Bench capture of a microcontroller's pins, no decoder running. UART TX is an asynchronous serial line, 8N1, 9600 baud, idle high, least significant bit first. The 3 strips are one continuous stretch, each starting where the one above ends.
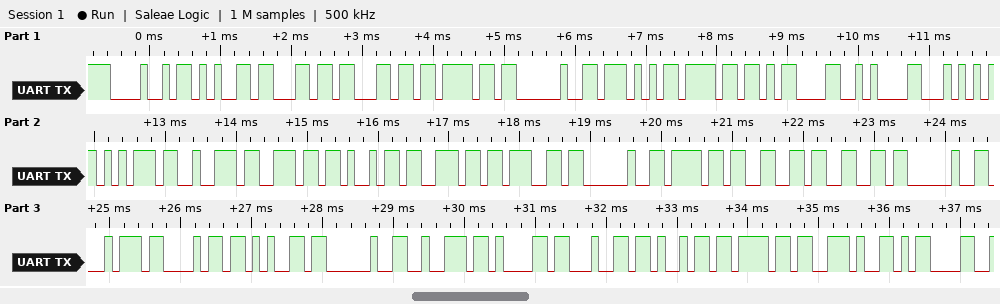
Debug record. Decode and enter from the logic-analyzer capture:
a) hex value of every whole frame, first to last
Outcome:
48 65 6C 6C 6F 20 57 6F 0D 0A 54 75 72 6E 69 6E 67 20 6F 66 66 20 74 68 65 20 72 61 64 69 6F 2E 0D
